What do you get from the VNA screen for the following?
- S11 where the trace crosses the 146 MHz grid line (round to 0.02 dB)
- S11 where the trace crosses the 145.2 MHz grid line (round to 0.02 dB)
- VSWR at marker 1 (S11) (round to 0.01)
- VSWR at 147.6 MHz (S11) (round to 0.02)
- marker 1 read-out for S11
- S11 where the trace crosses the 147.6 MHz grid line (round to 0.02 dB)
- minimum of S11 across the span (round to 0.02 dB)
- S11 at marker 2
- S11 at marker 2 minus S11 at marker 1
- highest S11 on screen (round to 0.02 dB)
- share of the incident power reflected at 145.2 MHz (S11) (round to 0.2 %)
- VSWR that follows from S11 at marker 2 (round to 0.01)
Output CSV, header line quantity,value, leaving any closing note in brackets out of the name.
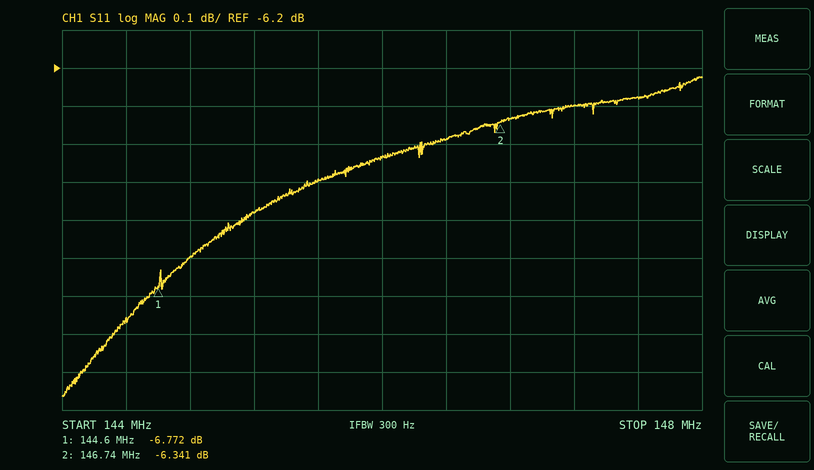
quantity,value
S11 where the trace crosses the 146 MHz grid line,-6.44 dB
S11 where the trace crosses the 145.2 MHz grid line,-6.58 dB
VSWR at marker 1 (S11),2.69
VSWR at 147.6 MHz (S11),2.88
marker 1 read-out for S11,-6.772 dB
S11 where the trace crosses the 147.6 MHz grid line,-6.28 dB
minimum of S11 across the span,-7.06 dB
S11 at marker 2,-6.341 dB
S11 at marker 2 minus S11 at marker 1,0.431 dB
highest S11 on screen,-6.22 dB
share of the incident power reflected at 145.2 MHz (S11),22.0 %
VSWR that follows from S11 at marker 2,2.86
